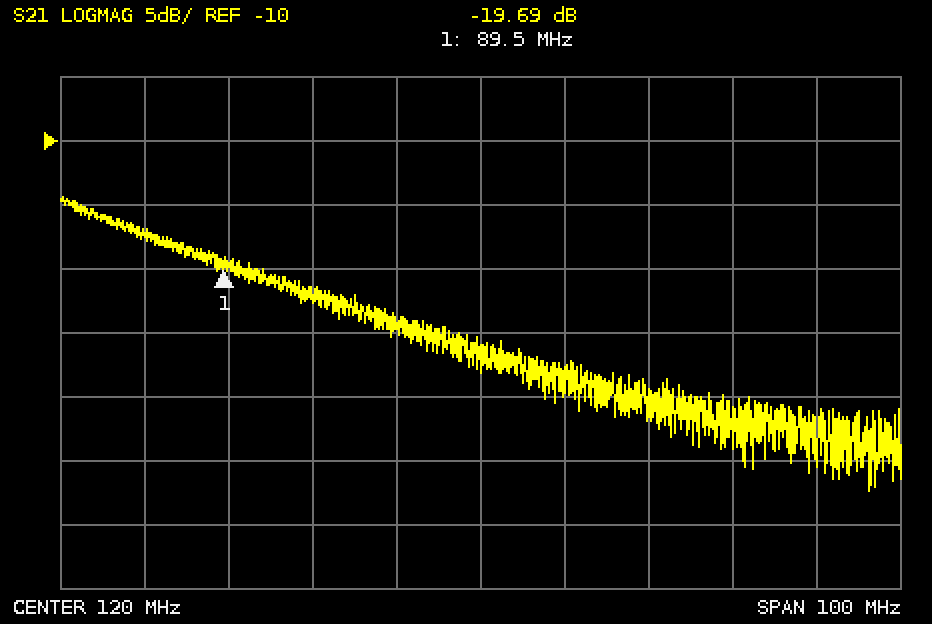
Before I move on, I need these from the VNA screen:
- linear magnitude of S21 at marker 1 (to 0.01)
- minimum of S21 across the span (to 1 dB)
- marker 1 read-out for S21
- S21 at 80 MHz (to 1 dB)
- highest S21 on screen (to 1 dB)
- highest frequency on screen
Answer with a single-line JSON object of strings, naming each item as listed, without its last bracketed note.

{"linear magnitude of S21 at marker 1": "0.10", "minimum of S21 across the span": "-37 dB", "marker 1 read-out for S21": "-19.69 dB", "S21 at 80 MHz": "-17 dB", "highest S21 on screen": "-14 dB", "highest frequency on screen": "170 MHz"}
